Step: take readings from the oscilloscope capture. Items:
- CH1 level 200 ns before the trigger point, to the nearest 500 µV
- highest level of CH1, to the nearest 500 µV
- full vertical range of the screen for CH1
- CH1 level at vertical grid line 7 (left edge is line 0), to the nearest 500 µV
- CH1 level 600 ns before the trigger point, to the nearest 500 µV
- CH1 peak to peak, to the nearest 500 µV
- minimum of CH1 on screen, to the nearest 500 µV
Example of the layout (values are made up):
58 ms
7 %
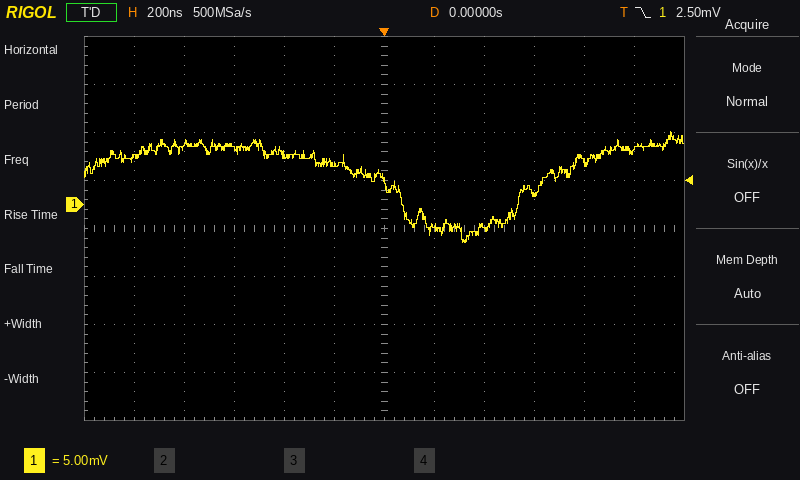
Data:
4.0 mV
7.5 mV
40 mV
-2.5 mV
6.0 mV
11.5 mV
-4.0 mV
